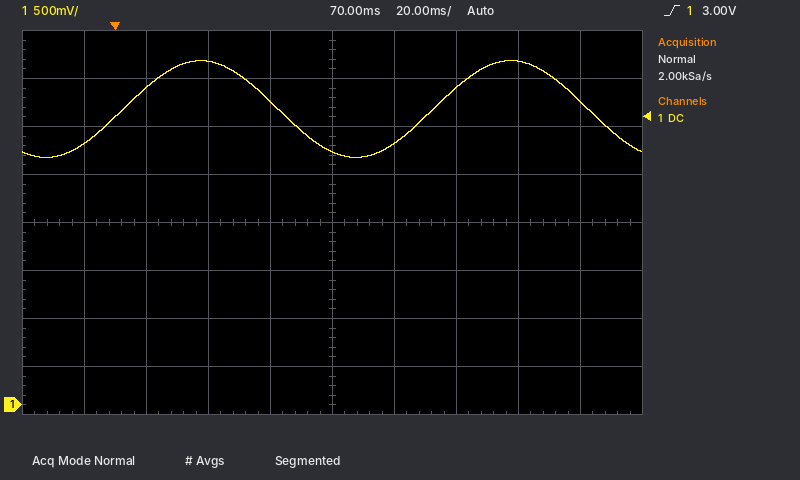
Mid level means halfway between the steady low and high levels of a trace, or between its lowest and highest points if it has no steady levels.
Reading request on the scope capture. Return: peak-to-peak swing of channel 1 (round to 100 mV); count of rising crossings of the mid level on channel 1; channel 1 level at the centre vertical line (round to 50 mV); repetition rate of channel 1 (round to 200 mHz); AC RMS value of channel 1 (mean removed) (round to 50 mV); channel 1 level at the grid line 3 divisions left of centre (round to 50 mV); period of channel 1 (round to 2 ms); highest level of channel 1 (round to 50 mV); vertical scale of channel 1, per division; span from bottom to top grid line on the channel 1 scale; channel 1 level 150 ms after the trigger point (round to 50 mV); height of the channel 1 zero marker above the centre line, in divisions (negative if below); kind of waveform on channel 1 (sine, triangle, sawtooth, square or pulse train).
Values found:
1.00 V
2
2.65 V
10.0 Hz
350 mV
3.30 V
100 ms
3.60 V
500 mV
4 V
3.15 V
-3.8 div
sine
